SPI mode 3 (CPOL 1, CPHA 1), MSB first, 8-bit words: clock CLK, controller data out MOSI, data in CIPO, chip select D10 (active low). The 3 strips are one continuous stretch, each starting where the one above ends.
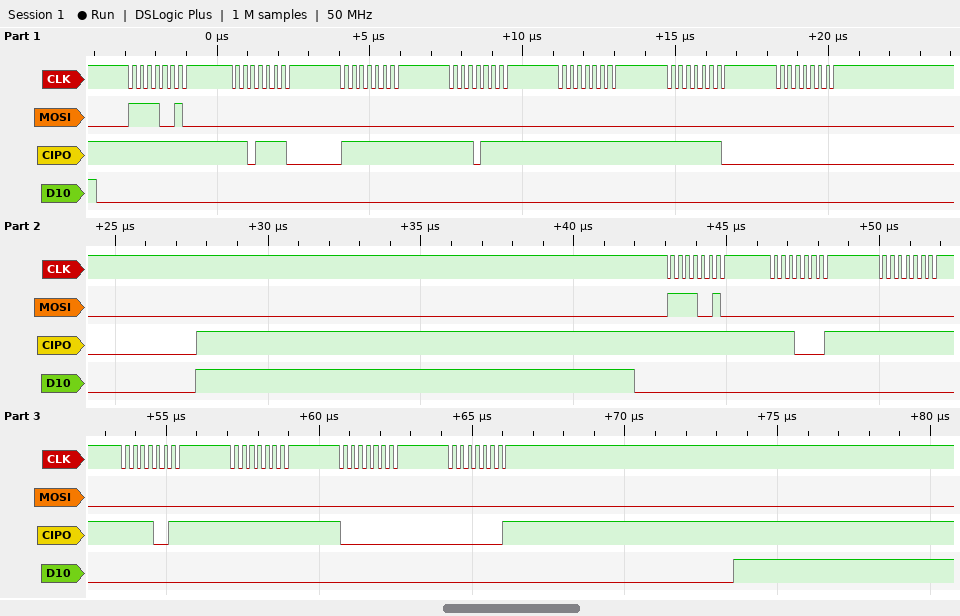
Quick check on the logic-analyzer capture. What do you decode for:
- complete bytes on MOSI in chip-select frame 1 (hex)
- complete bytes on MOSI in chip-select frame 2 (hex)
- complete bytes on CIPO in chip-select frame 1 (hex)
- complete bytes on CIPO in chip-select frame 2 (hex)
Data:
F2 00 00 00 00 00 00
F2 00 00 00 00 00 00
FF DE FF EF FF FE 00
FF E1 FF F3 FF 00 01
